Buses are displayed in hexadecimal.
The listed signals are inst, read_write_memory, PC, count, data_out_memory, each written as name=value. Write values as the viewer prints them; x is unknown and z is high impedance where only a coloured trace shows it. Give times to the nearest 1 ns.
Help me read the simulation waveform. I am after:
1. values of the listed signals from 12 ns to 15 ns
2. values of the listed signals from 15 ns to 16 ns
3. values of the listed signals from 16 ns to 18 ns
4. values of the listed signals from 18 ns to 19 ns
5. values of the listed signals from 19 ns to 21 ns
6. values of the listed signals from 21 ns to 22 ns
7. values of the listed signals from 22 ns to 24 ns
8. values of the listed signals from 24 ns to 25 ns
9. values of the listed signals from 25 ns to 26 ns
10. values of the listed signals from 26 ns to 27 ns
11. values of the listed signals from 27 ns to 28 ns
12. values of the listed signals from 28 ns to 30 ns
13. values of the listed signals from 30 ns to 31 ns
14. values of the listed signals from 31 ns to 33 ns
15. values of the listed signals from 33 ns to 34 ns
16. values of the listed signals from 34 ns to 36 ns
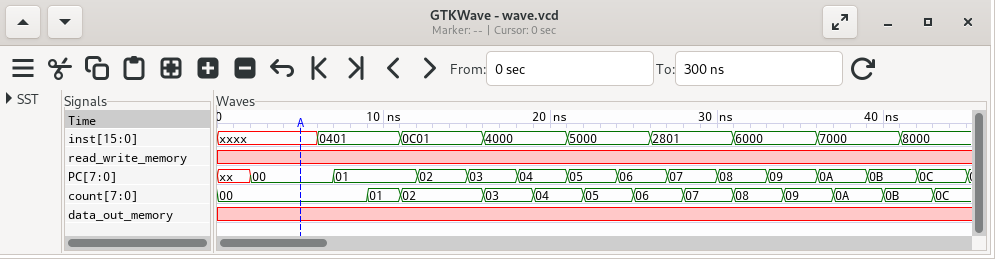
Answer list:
inst=0C01, read_write_memory=x, PC=02, count=02, data_out_memory=x
inst=0C01, read_write_memory=x, PC=03, count=02, data_out_memory=x
inst=4000, read_write_memory=x, PC=03, count=03, data_out_memory=x
inst=4000, read_write_memory=x, PC=04, count=03, data_out_memory=x
inst=4000, read_write_memory=x, PC=04, count=04, data_out_memory=x
inst=5000, read_write_memory=x, PC=05, count=04, data_out_memory=x
inst=5000, read_write_memory=x, PC=05, count=05, data_out_memory=x
inst=5000, read_write_memory=x, PC=06, count=05, data_out_memory=x
inst=5000, read_write_memory=x, PC=06, count=06, data_out_memory=x
inst=2801, read_write_memory=x, PC=06, count=06, data_out_memory=x
inst=2801, read_write_memory=x, PC=07, count=06, data_out_memory=x
inst=2801, read_write_memory=x, PC=07, count=07, data_out_memory=x
inst=2801, read_write_memory=x, PC=08, count=07, data_out_memory=x
inst=6000, read_write_memory=x, PC=08, count=08, data_out_memory=x
inst=6000, read_write_memory=x, PC=09, count=08, data_out_memory=x
inst=6000, read_write_memory=x, PC=09, count=09, data_out_memory=x
